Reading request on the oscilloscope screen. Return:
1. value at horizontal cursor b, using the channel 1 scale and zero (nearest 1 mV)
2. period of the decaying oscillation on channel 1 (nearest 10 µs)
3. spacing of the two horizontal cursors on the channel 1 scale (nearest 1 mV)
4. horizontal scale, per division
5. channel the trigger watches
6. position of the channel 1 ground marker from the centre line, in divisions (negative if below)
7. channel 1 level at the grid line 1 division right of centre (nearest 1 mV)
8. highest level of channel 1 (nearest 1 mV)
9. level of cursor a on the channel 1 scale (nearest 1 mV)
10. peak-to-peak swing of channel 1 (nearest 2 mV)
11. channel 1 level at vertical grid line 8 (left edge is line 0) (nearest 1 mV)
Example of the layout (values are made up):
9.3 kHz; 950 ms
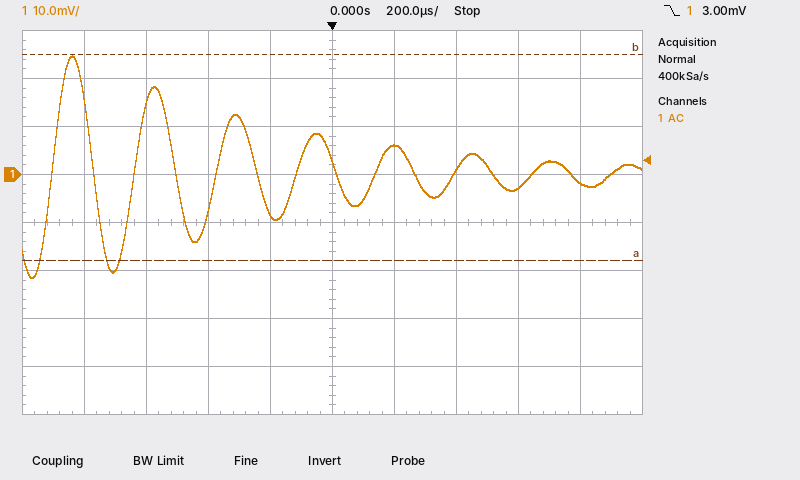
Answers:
25 mV; 260 µs; 43 mV; 200 µs; channel 1; +1.0 div; 6 mV; 25 mV; -18 mV; 46 mV; -3 mV
